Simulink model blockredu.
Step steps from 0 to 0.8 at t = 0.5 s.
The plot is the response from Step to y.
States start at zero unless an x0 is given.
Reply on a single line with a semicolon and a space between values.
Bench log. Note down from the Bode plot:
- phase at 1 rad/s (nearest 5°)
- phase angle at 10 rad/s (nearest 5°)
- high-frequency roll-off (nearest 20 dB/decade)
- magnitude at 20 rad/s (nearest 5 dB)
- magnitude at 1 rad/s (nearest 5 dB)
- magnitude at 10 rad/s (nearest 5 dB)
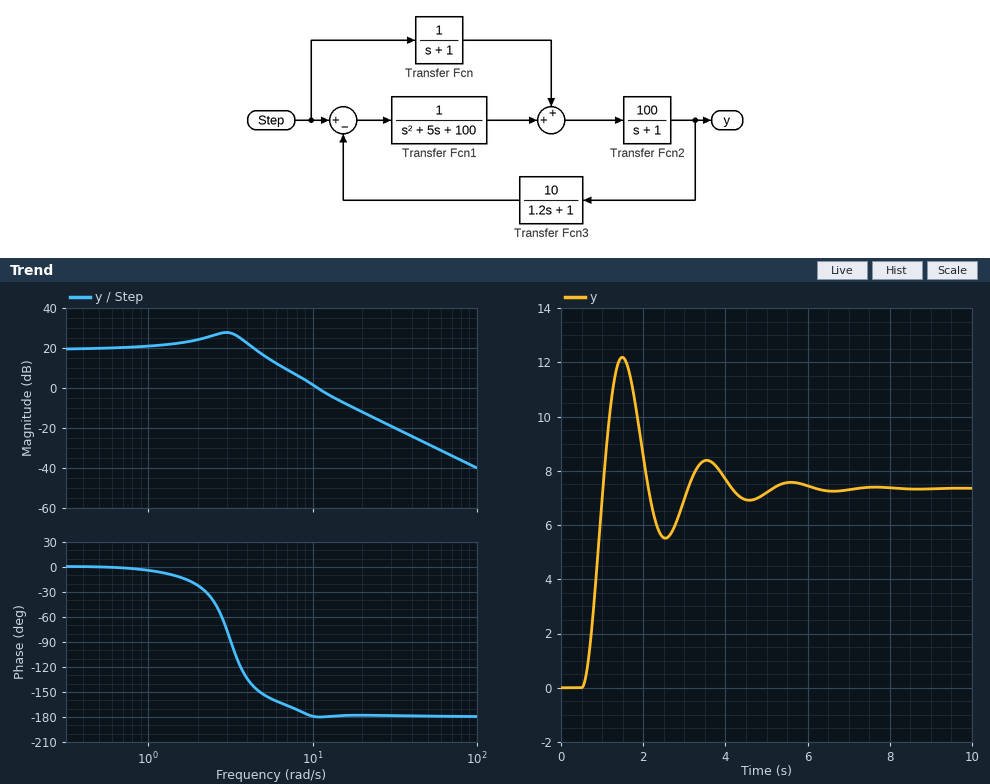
-5°; -180°; -40 dB/decade; -10 dB; 20 dB; 0 dB
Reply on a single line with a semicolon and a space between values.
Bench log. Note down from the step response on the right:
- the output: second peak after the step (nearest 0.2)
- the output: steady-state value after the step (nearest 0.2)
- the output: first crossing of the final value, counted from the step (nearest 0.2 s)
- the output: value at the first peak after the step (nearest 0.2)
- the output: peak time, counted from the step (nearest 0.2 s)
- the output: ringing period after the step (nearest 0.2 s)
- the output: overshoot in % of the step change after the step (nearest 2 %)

8.4; 7.4; 0.6 s; 12.2; 1.0 s; 2.0 s; 66 %
